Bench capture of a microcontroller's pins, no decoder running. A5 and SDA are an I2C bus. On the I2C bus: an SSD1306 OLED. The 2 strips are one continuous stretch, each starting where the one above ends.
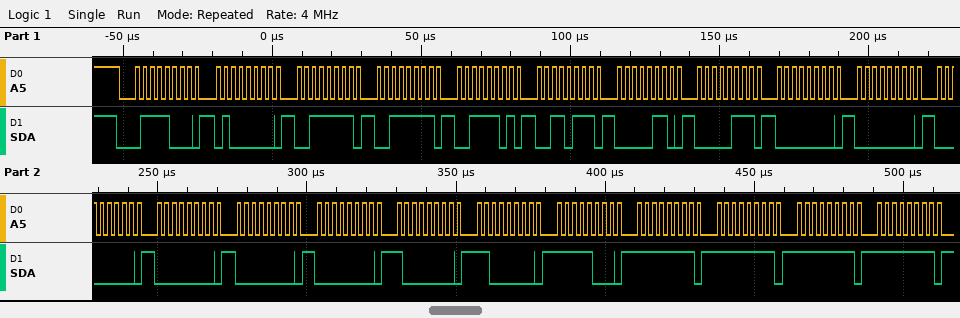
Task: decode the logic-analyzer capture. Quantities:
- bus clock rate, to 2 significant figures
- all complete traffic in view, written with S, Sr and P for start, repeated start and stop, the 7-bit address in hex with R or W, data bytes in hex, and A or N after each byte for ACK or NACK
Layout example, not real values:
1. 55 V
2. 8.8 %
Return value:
1. 400 kHz
2. S 3CW A 40 A 3F A 3F A 3D A 37 A 06 A 07 A 00 A 00 A 00 A 00 A 00 A 00 A 80 A C0 A F8 A FF A FF A FF A FF A
